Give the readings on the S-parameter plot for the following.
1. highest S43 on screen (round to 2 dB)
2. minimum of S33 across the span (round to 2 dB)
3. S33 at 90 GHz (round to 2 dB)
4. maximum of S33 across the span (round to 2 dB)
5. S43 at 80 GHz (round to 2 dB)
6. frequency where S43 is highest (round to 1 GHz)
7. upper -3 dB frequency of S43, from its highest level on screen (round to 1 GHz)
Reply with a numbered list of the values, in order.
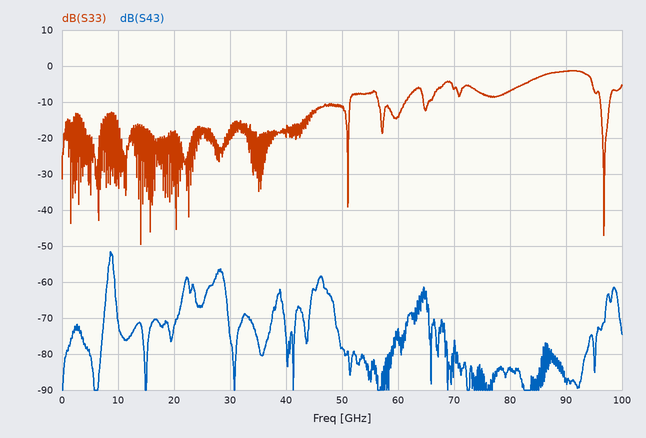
1. -52 dB
2. -50 dB
3. -2 dB
4. -2 dB
5. -84 dB
6. 9 GHz
7. 9 GHz
